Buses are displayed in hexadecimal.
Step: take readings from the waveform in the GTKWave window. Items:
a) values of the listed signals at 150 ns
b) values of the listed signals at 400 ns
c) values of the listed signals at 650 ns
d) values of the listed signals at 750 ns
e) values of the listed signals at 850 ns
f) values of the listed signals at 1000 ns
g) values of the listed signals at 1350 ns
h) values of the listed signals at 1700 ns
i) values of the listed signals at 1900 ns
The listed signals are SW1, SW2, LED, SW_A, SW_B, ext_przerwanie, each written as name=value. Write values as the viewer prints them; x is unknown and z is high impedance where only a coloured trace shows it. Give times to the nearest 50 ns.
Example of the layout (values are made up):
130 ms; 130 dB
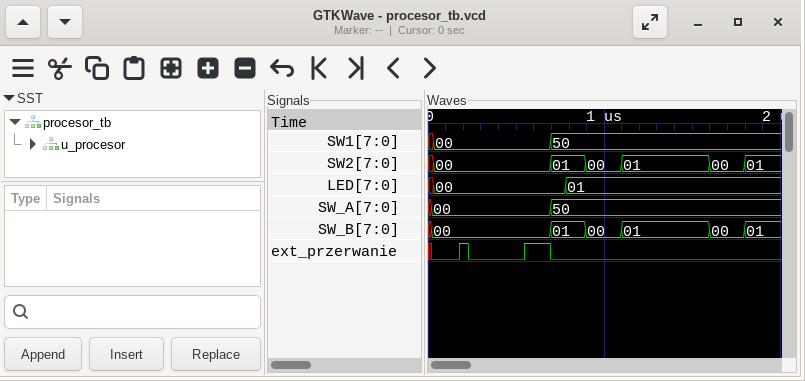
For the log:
SW1=00, SW2=00, LED=00, SW_A=00, SW_B=00, ext_przerwanie=0; SW1=00, SW2=00, LED=00, SW_A=00, SW_B=00, ext_przerwanie=0; SW1=00, SW2=00, LED=00, SW_A=00, SW_B=00, ext_przerwanie=1; SW1=50, SW2=01, LED=00, SW_A=50, SW_B=01, ext_przerwanie=0; SW1=50, SW2=01, LED=01, SW_A=50, SW_B=01, ext_przerwanie=0; SW1=50, SW2=00, LED=01, SW_A=50, SW_B=00, ext_przerwanie=0; SW1=50, SW2=01, LED=01, SW_A=50, SW_B=01, ext_przerwanie=0; SW1=50, SW2=00, LED=01, SW_A=50, SW_B=00, ext_przerwanie=0; SW1=50, SW2=01, LED=01, SW_A=50, SW_B=01, ext_przerwanie=0
